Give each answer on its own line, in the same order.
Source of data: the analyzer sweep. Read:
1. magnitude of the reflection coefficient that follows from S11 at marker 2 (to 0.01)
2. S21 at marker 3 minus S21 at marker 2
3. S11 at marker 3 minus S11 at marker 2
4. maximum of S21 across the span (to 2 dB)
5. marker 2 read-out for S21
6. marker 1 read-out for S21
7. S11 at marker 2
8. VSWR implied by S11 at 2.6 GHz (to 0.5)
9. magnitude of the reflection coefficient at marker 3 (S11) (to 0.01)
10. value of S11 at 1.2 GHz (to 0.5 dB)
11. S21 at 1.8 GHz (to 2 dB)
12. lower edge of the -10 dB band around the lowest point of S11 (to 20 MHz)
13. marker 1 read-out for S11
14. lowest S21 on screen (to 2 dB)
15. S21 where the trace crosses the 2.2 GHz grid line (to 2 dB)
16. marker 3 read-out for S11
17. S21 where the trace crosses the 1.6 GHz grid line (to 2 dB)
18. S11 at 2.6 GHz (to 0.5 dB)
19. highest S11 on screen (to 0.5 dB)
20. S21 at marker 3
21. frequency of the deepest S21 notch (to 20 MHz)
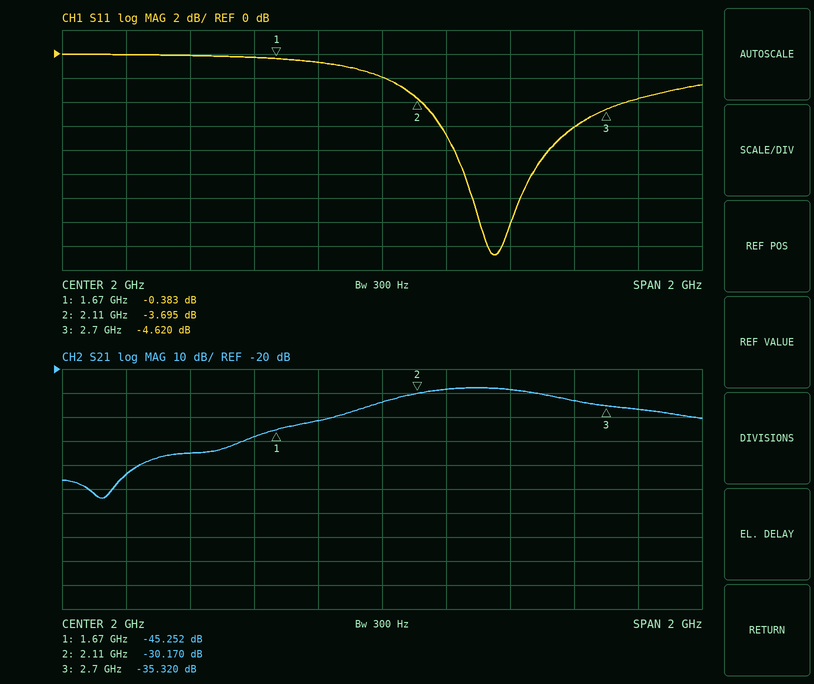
0.65
-5.150 dB
-0.925 dB
-28 dB
-30.170 dB
-45.252 dB
-3.695 dB
3.0
0.59
0.0 dB
-42 dB
2.26 GHz
-0.383 dB
-74 dB
-28 dB
-4.620 dB
-48 dB
-6.0 dB
0.0 dB
-35.320 dB
1.12 GHz
